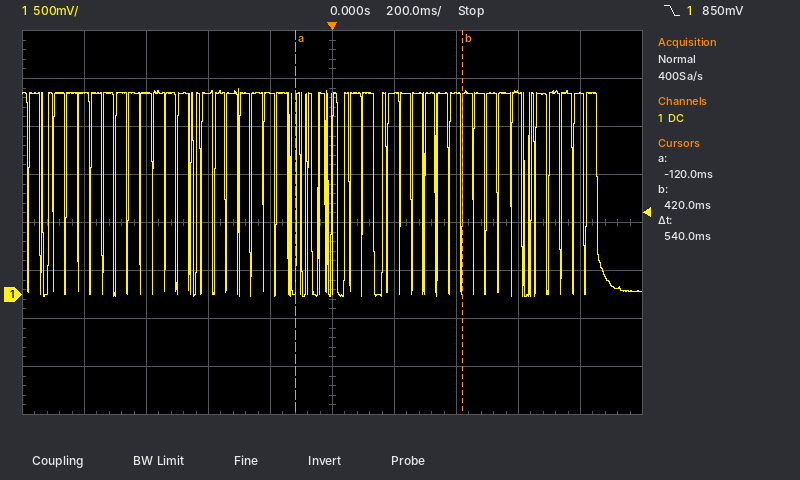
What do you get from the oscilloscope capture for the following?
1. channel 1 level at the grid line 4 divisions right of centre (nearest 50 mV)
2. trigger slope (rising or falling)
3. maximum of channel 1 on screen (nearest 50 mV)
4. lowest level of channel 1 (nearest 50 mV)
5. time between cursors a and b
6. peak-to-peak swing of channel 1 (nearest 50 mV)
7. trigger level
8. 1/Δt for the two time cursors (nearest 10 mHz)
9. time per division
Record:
2.10 V
falling
2.15 V
0 mV
540 ms
2.15 V
850 mV
1.85 Hz
200 ms
